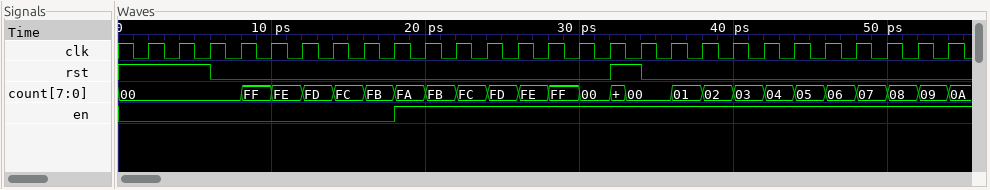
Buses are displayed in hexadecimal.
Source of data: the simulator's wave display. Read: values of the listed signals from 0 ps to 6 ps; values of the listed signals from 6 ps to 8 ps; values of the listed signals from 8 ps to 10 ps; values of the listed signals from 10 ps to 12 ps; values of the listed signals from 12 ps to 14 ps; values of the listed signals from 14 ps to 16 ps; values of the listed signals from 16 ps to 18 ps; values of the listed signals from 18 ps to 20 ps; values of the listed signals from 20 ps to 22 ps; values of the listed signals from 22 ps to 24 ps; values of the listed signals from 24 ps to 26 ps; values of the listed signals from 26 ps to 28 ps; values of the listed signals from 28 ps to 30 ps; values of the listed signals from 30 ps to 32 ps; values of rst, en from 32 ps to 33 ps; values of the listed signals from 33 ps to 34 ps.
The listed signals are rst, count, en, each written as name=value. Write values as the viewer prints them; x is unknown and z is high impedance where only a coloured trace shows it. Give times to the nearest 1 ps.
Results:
rst=1, count=00, en=0
rst=0, count=00, en=0
rst=0, count=FF, en=0
rst=0, count=FE, en=0
rst=0, count=FD, en=0
rst=0, count=FC, en=0
rst=0, count=FB, en=0
rst=0, count=FA, en=1
rst=0, count=FB, en=1
rst=0, count=FC, en=1
rst=0, count=FD, en=1
rst=0, count=FE, en=1
rst=0, count=FF, en=1
rst=0, count=00, en=1
rst=1, en=1
rst=1, count=00, en=1
